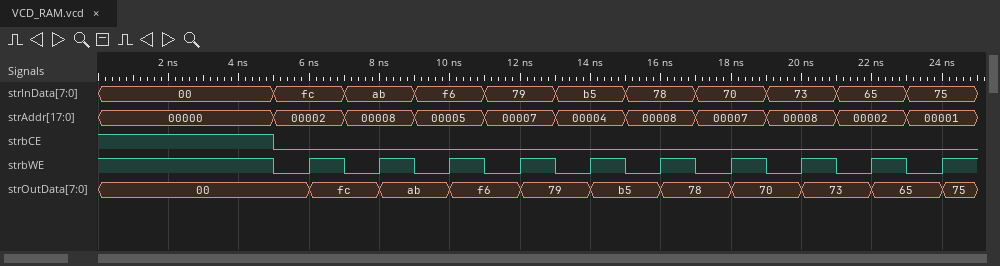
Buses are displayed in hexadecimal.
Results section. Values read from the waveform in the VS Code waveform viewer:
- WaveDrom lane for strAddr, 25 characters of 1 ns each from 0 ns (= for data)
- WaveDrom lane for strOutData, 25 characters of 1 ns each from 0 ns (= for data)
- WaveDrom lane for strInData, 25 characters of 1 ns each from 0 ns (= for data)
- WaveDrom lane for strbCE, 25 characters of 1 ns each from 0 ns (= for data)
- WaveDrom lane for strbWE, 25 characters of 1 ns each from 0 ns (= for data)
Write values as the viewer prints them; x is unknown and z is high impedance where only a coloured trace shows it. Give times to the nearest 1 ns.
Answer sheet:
{name: 'strAddr', wave: '=....=.=.=.=.=.=.=.=.=.=.', data: '00000 00002 00008 00005 00007 00004 00008 00007 00008 00002 00001'}
{name: 'strOutData', wave: '=.....=.=.=.=.=.=.=.=.=.=', data: '00 fc ab f6 79 b5 78 70 73 65 75'}
{name: 'strInData', wave: '=....=.=.=.=.=.=.=.=.=.=.', data: '00 fc ab f6 79 b5 78 70 73 65 75'}
{name: 'strbCE', wave: '1....0...................'}
{name: 'strbWE', wave: '1....01010101010101010101'}
